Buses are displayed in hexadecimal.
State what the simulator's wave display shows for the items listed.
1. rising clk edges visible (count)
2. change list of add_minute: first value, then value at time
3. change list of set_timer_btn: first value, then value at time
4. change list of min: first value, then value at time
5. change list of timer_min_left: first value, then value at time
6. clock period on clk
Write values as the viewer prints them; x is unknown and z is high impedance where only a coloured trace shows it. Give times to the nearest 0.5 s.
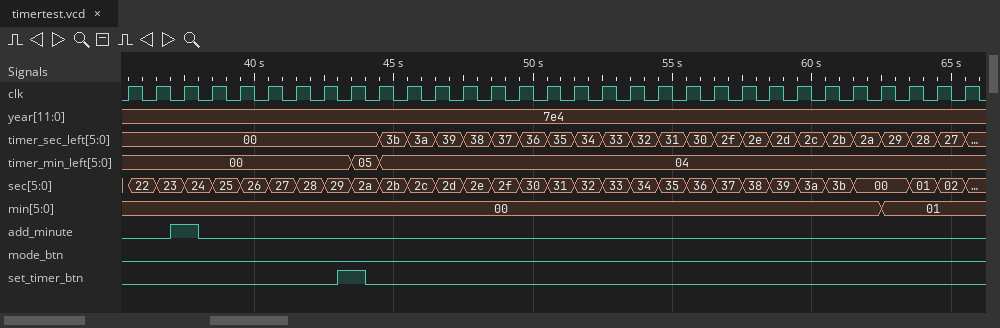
31
0, 1 at 37 s, 0 at 38 s
0, 1 at 43 s, 0 at 44 s
00, 01 at 62.5 s
00, 05 at 43.5 s, 04 at 44.5 s
1 s
